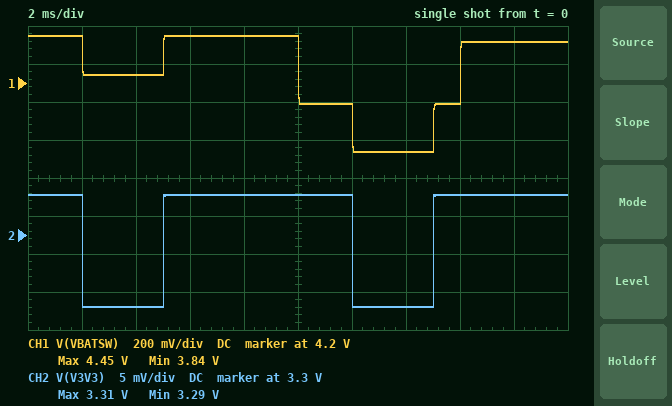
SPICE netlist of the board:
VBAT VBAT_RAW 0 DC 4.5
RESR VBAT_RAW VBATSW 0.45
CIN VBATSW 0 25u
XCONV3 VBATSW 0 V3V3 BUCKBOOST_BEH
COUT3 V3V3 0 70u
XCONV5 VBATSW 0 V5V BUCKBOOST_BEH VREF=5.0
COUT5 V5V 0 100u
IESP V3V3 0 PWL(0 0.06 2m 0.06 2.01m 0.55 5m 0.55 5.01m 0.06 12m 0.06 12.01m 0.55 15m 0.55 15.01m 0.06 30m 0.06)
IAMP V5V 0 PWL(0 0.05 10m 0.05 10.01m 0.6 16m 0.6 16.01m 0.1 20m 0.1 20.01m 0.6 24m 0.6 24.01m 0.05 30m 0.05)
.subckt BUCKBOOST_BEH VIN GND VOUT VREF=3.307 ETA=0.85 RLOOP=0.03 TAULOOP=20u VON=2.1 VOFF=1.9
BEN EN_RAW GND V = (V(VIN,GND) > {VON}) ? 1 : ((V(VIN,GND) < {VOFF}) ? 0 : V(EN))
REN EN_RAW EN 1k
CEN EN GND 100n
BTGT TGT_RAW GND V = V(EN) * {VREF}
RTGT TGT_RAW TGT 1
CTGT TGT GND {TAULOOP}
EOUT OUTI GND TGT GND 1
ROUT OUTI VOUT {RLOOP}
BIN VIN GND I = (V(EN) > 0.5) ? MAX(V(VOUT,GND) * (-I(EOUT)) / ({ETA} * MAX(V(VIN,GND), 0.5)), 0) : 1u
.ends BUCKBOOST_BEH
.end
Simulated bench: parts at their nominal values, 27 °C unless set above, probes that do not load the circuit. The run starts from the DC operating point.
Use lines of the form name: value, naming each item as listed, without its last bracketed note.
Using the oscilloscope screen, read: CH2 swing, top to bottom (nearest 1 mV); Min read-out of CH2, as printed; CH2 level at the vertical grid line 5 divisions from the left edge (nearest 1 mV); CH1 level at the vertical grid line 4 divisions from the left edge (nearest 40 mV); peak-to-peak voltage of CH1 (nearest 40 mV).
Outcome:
CH2 swing, top to bottom: 15 mV
Min read-out of CH2, as printed: 3.29 V
CH2 level at the vertical grid line 5 divisions from the left edge: 3.305 V
CH1 level at the vertical grid line 4 divisions from the left edge: 4.44 V
peak-to-peak voltage of CH1: 600 mV
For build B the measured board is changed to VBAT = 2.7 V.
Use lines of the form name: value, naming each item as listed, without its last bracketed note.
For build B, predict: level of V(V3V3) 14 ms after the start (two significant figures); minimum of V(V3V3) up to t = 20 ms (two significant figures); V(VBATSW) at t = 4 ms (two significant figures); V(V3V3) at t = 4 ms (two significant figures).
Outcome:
level of V(V3V3) 14 ms after the start: 1.8 V
minimum of V(V3V3) up to t = 20 ms: 1.7 V
V(VBATSW) at t = 4 ms: 2.2 V
V(V3V3) at t = 4 ms: 3.3 V
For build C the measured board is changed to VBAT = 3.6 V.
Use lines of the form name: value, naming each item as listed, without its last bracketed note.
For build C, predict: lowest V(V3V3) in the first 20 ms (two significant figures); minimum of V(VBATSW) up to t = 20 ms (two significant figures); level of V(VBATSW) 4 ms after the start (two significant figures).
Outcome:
lowest V(V3V3) in the first 20 ms: 3.3 V
minimum of V(VBATSW) up to t = 20 ms: 2.6 V
level of V(VBATSW) 4 ms after the start: 3.3 V
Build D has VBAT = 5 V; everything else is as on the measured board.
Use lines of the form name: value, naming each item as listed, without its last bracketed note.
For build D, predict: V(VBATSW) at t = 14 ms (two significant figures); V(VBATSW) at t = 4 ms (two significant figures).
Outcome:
V(VBATSW) at t = 14 ms: 4.4 V
V(VBATSW) at t = 4 ms: 4.8 V
